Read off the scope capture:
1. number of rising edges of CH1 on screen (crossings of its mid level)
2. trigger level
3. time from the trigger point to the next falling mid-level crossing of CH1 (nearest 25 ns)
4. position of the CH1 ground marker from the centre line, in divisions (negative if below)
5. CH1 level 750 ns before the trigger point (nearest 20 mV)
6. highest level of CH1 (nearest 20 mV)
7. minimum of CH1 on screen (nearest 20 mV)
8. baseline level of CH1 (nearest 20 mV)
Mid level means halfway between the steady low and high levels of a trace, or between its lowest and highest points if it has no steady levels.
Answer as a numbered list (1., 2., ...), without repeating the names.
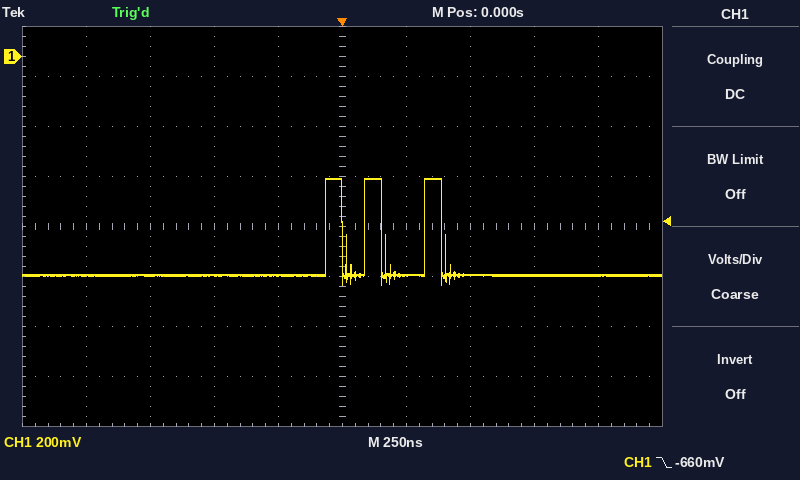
1. 3
2. -660 mV
3. 150 ns
4. +3.4 div
5. -880 mV
6. -480 mV
7. -920 mV
8. -880 mV
